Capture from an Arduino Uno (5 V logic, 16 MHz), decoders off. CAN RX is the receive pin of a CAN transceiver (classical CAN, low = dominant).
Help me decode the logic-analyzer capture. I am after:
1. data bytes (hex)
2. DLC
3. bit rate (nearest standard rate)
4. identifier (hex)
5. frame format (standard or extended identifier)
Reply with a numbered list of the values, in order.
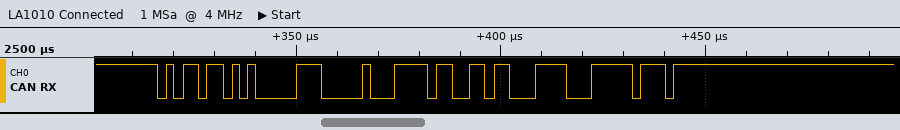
1. 00 F6 6C
2. 3
3. 500 kbit/s
4. 0x5B5
5. standard
